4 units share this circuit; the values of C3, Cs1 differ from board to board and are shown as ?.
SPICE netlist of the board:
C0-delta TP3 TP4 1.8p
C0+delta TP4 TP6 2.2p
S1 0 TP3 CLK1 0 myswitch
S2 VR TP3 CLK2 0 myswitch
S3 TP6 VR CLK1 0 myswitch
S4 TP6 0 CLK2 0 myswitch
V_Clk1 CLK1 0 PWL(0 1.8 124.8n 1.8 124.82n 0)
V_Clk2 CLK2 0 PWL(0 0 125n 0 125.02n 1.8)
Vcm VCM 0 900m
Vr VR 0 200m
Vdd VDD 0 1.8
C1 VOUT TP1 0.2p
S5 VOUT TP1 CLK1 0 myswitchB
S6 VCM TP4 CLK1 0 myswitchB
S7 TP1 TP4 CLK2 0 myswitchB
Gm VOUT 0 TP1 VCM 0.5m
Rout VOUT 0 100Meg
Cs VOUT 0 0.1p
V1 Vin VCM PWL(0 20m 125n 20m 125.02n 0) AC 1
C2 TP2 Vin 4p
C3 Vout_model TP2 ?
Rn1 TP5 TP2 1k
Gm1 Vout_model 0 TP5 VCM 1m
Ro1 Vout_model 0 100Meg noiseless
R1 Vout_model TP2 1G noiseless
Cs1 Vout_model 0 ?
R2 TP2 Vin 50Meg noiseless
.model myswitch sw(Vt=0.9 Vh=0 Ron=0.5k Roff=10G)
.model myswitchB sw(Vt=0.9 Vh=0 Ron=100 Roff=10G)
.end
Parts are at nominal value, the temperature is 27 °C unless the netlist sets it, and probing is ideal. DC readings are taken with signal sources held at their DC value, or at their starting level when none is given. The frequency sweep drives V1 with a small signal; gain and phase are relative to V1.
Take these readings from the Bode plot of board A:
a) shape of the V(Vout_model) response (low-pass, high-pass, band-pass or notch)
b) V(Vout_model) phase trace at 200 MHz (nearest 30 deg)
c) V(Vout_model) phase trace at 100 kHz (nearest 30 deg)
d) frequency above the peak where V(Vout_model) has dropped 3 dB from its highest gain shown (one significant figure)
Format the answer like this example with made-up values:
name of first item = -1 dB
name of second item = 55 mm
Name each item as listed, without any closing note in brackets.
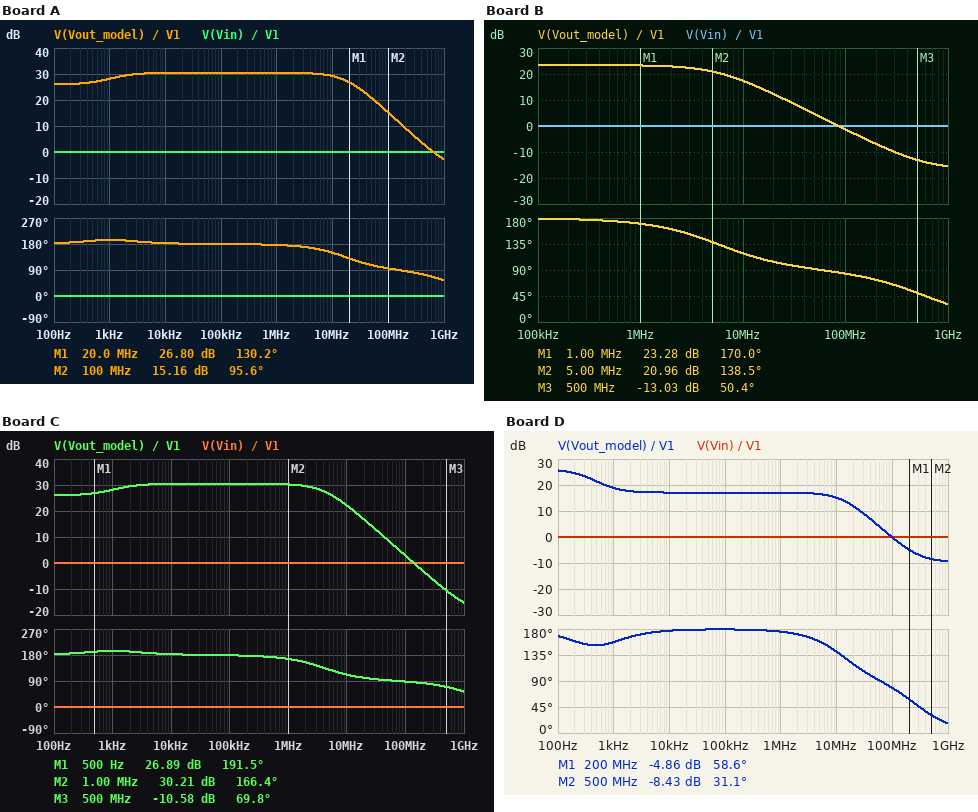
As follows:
shape of the V(Vout_model) response = low-pass
V(Vout_model) phase trace at 200 MHz = 90 deg
V(Vout_model) phase trace at 100 kHz = 180 deg
frequency above the peak where V(Vout_model) has dropped 3 dB from its highest gain shown = 20 MHz
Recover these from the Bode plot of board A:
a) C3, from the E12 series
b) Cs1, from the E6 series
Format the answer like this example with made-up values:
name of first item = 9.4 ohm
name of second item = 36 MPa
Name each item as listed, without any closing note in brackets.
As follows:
C3, from the E12 series = 120 fF
Cs1, from the E6 series = 150 fF
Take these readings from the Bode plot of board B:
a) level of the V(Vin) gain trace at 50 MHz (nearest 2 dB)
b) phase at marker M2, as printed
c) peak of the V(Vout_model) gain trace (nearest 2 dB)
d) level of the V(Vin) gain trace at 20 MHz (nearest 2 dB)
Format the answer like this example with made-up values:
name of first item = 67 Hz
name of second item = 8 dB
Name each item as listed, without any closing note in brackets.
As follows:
level of the V(Vin) gain trace at 50 MHz = 0 dB
phase at marker M2, as printed = 138.5 deg
peak of the V(Vout_model) gain trace = 24 dB
level of the V(Vin) gain trace at 20 MHz = 0 dB
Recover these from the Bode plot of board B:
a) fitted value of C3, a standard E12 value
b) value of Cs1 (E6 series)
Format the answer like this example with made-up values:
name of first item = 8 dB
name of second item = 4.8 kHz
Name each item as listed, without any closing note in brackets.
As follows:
fitted value of C3, a standard E12 value = 270 fF
value of Cs1 = 1.5 pF
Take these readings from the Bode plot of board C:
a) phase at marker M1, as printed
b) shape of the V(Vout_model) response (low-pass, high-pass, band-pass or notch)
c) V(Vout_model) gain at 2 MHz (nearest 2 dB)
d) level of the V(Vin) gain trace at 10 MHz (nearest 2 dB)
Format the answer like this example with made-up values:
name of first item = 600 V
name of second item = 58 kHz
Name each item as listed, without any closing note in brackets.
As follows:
phase at marker M1, as printed = 191.5 deg
shape of the V(Vout_model) response = low-pass
V(Vout_model) gain at 2 MHz = 30 dB
level of the V(Vin) gain trace at 10 MHz = 0 dB
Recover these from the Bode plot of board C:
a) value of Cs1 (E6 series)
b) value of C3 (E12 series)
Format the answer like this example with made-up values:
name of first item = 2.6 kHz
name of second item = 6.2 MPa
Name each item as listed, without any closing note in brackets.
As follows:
value of Cs1 = 1 pF
value of C3 = 120 fF
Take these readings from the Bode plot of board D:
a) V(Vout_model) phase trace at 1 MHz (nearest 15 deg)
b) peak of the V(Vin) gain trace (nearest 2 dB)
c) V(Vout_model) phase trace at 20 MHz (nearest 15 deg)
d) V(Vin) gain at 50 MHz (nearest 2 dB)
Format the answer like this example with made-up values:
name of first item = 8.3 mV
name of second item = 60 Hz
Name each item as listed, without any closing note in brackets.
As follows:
V(Vout_model) phase trace at 1 MHz = 180 deg
peak of the V(Vin) gain trace = 0 dB
V(Vout_model) phase trace at 20 MHz = 120 deg
V(Vin) gain at 50 MHz = 0 dB
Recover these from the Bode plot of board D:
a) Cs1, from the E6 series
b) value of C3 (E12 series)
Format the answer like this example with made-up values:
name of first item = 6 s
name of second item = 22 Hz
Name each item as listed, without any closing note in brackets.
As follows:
Cs1, from the E6 series = 1 pF
value of C3 = 560 fF
